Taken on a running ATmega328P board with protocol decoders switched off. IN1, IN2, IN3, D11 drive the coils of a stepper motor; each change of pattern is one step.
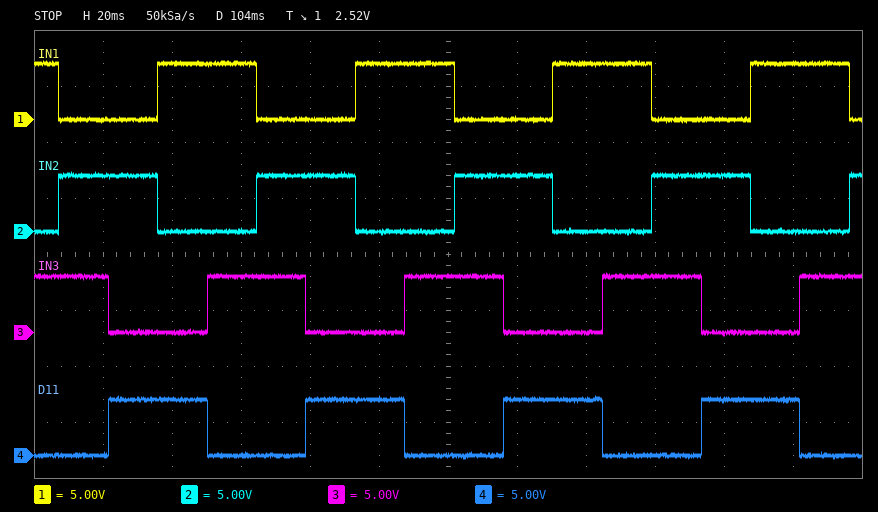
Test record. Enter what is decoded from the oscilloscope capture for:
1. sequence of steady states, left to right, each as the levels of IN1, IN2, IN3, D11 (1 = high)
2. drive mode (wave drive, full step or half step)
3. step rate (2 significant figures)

1010 0110 0101 1001 1010 0110 0101 1001 1010 0110 0101 1001 1010 0110 0101 1001 1010 0110
full step
70 steps/s
